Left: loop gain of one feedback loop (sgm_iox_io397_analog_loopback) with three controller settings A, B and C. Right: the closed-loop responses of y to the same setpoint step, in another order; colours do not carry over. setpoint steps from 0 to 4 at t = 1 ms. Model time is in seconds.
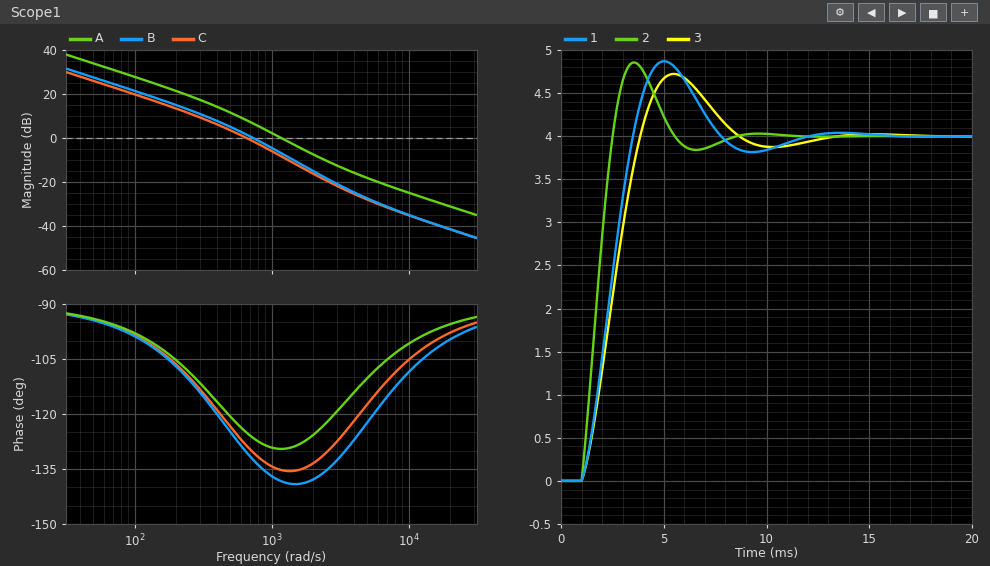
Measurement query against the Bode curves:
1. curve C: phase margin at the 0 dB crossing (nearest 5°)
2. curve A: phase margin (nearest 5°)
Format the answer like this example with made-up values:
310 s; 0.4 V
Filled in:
50°; 50°
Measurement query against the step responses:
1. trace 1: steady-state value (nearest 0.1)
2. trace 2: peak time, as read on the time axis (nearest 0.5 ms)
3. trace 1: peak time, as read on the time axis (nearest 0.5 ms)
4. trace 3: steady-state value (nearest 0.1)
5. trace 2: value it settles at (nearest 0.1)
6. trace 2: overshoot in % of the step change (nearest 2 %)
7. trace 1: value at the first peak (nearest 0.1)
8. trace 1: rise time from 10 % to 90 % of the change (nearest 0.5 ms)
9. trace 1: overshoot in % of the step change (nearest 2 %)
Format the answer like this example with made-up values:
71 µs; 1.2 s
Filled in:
4.0; 3.5 ms; 5.0 ms; 4.0; 4.0; 22 %; 4.9; 2.0 ms; 22 %
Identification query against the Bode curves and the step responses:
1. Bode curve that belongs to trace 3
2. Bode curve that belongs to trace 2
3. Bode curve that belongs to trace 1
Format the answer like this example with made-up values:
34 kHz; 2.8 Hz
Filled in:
C; A; B
